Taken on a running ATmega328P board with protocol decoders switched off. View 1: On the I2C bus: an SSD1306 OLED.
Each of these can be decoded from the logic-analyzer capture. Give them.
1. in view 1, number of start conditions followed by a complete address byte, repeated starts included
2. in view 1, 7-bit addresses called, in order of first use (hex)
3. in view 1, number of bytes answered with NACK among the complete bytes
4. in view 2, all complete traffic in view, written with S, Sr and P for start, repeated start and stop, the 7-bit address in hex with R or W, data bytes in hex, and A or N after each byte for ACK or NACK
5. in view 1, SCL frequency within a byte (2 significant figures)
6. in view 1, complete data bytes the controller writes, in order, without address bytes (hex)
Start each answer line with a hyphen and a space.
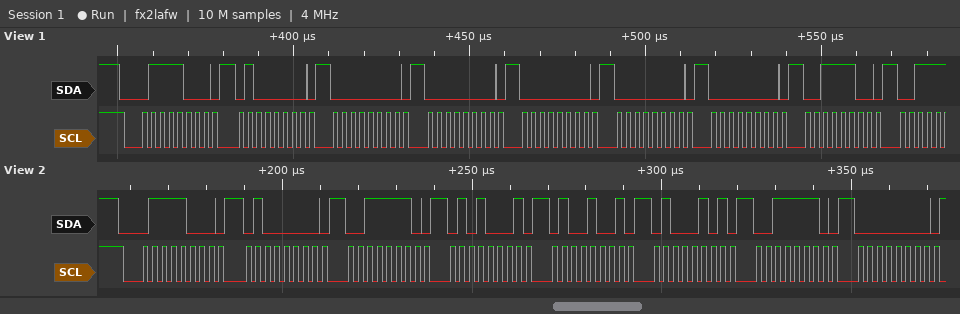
- 1
- 0x3C
- 0
- S 3CW A 40 A 3E A 51 A 49 A 45 A 3E A 00 A
- 400 kHz
- 40 00 00 00 00 00 3C
